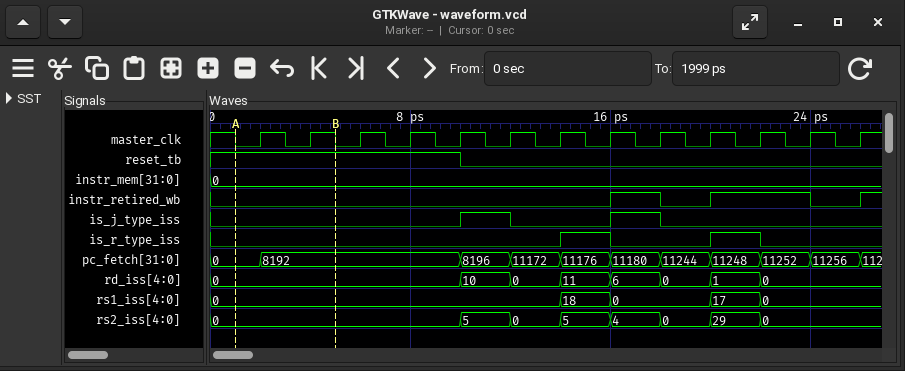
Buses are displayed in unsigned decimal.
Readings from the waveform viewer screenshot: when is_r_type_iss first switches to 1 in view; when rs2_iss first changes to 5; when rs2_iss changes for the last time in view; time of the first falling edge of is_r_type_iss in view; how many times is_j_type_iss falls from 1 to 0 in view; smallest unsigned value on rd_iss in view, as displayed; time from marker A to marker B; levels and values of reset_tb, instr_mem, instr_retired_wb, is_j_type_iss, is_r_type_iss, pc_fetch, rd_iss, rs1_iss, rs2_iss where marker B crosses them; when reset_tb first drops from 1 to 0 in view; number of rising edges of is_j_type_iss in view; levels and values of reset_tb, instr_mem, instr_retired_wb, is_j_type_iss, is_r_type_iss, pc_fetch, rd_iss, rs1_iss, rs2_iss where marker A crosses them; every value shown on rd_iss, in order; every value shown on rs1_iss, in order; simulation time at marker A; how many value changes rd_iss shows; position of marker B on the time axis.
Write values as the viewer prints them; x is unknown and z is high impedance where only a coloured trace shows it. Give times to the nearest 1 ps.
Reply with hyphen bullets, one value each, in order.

- 14 ps
- 10 ps
- 22 ps
- 16 ps
- 2
- 0
- 4 ps
- reset_tb=1, instr_mem=0, instr_retired_wb=0, is_j_type_iss=0, is_r_type_iss=0, pc_fetch=8192, rd_iss=0, rs1_iss=0, rs2_iss=0
- 10 ps
- 2
- reset_tb=1, instr_mem=0, instr_retired_wb=0, is_j_type_iss=0, is_r_type_iss=0, pc_fetch=0, rd_iss=0, rs1_iss=0, rs2_iss=0
- 0, 10, 0, 11, 6, 0, 1, 0
- 0, 18, 0, 17, 0
- 1 ps
- 7
- 5 ps
